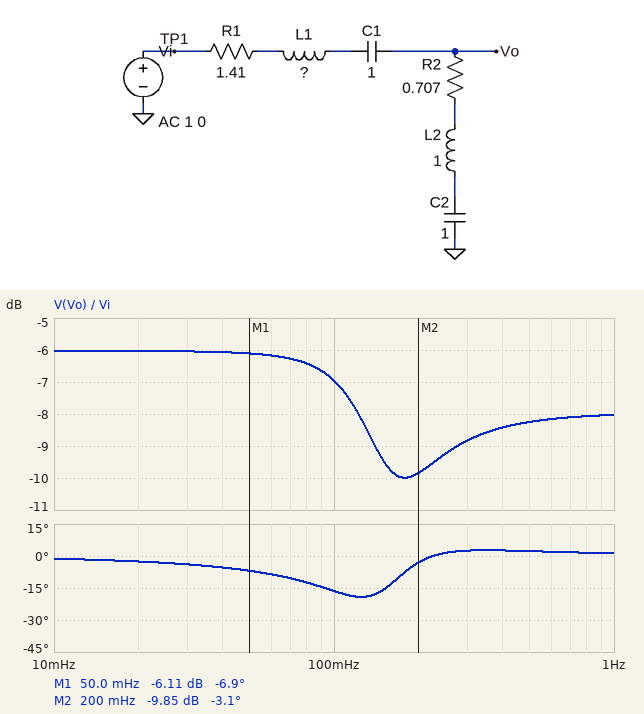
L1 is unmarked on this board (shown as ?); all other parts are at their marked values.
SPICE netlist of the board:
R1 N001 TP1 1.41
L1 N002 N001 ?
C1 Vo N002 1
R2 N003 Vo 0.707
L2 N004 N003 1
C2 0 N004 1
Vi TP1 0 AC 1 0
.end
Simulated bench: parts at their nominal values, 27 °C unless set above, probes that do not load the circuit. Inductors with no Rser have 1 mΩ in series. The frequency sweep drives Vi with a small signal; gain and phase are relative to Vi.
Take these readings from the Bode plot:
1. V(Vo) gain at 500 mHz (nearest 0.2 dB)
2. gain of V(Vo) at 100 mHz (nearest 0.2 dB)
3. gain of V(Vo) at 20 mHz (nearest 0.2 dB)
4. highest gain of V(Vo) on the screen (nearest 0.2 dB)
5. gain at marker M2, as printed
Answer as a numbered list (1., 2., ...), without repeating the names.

1. -8.2 dB
2. -7.0 dB
3. -6.0 dB
4. -6.0 dB
5. -9.85 dB
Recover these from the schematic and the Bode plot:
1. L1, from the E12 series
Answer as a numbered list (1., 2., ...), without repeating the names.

1. 1.5 H
